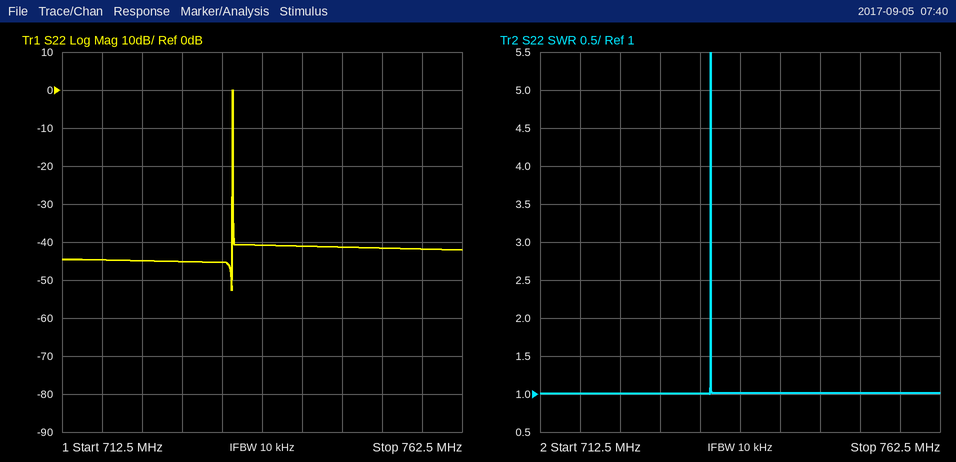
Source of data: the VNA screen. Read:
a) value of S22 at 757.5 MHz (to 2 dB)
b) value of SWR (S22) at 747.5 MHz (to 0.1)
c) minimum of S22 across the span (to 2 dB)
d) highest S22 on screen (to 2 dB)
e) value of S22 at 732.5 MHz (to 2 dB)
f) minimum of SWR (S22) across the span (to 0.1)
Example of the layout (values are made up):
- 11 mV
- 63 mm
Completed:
- -42 dB
- 1.0
- -52 dB
- 0 dB
- -46 dB
- 1.0
